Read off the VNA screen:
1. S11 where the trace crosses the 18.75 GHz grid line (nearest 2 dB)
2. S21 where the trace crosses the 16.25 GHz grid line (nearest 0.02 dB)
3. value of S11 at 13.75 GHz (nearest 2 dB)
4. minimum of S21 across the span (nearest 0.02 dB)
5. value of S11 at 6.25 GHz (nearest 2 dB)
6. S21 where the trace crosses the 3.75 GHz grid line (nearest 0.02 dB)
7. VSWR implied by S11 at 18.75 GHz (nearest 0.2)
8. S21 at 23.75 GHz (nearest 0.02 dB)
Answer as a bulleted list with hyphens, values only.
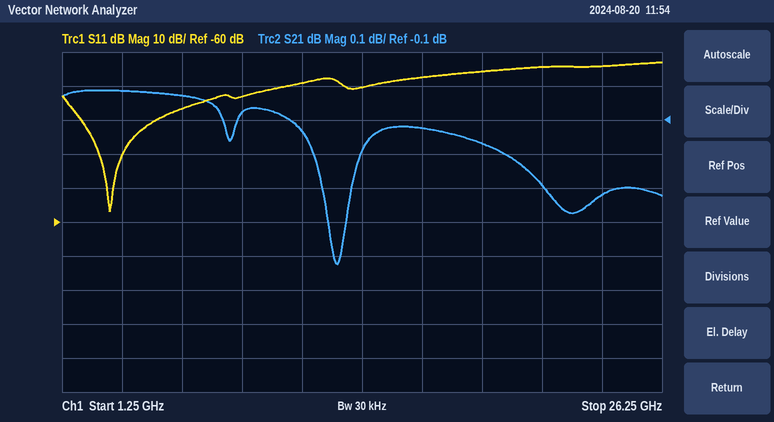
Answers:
- -16 dB
- -0.12 dB
- -20 dB
- -0.52 dB
- -26 dB
- -0.02 dB
- 1.4
- -0.32 dB
